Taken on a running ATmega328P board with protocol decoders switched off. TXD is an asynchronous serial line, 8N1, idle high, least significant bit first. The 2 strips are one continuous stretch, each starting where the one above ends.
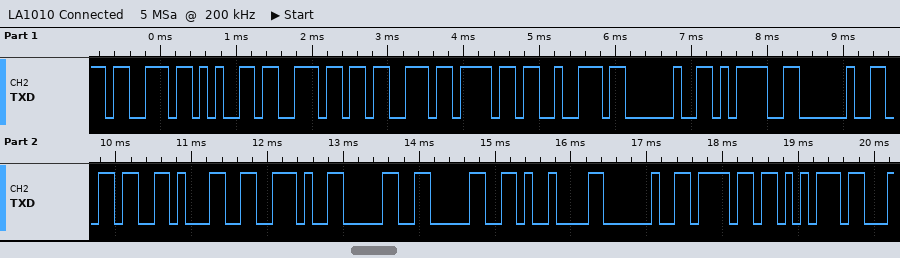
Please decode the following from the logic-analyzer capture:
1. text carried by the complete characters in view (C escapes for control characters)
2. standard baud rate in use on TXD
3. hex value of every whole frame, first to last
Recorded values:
"sensor = 61.00\t ou"
9600 baud
0x73 0x65 0x6E 0x73 0x6F 0x72 0x20 0x3D 0x20 0x36 0x31 0x2E 0x30 0x30 0x09 0x20 0x6F 0x75
